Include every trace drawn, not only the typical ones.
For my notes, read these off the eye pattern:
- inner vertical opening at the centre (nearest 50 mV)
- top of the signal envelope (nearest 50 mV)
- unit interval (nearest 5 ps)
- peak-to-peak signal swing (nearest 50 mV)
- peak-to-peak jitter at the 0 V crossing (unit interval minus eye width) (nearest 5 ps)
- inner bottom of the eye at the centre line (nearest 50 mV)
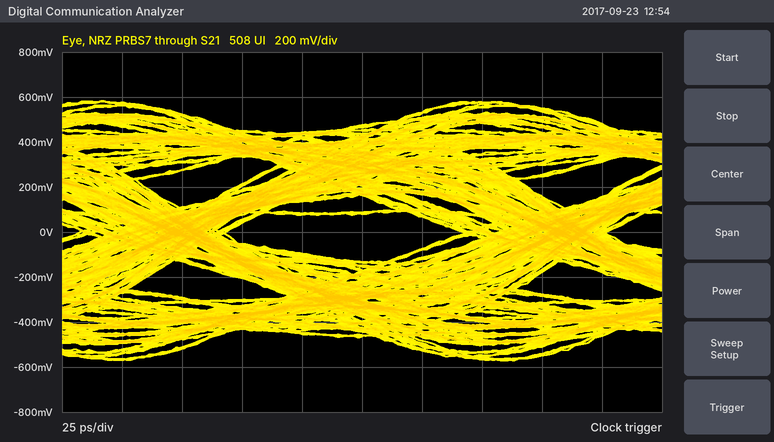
200 mV
600 mV
160 ps
1.15 V
60 ps
-150 mV
